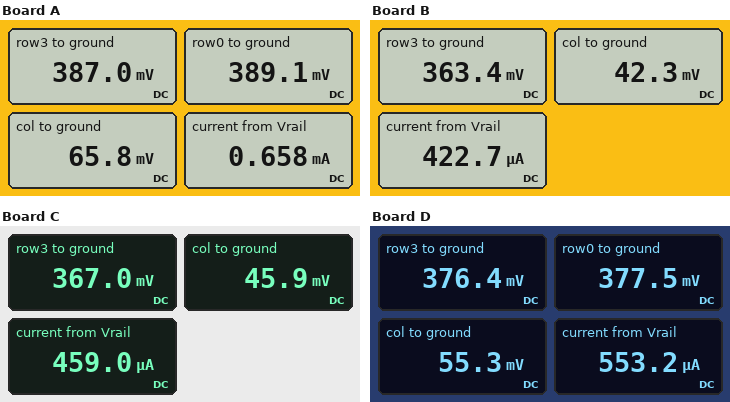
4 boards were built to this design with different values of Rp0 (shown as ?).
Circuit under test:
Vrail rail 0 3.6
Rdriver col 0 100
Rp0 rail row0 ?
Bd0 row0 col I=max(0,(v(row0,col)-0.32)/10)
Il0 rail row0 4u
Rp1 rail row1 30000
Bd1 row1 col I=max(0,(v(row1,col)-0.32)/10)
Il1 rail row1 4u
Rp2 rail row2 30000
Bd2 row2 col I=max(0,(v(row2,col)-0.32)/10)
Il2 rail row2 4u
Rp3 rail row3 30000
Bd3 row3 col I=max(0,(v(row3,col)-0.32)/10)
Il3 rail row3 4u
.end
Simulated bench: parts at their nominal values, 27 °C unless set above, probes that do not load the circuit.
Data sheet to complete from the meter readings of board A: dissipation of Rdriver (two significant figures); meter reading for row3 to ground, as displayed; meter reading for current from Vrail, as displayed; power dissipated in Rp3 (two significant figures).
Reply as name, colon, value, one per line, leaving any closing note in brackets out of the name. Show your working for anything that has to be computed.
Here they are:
dissipation of Rdriver: (65.8 mV)^2 / 100 Ω = 43 µW
meter reading for row3 to ground, as displayed: 387.0 mV
meter reading for current from Vrail, as displayed: 0.658 mA
power dissipated in Rp3: (3.6 V - 387 mV)^2 / 30 kΩ = 340 µW
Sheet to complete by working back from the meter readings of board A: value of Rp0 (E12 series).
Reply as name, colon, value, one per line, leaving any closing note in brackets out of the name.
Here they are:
value of Rp0: 10 kΩ
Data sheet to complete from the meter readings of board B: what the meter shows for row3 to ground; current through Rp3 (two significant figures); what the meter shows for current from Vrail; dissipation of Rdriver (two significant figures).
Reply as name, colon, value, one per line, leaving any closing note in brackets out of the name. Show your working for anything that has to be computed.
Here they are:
what the meter shows for row3 to ground: 363.4 mV
current through Rp3: (3.6 V - 363.4 mV) / 30 kΩ = 110 µA
what the meter shows for current from Vrail: 422.7 µA
dissipation of Rdriver: (42.3 mV)^2 / 100 Ω = 18 µW
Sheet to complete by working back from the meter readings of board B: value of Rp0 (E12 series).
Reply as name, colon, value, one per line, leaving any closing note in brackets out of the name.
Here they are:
value of Rp0: 39 kΩ
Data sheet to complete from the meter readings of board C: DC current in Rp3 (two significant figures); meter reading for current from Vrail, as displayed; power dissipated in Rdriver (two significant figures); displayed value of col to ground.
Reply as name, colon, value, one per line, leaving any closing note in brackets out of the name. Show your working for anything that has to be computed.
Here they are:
DC current in Rp3: (3.6 V - 367 mV) / 30 kΩ = 110 µA
meter reading for current from Vrail, as displayed: 459.0 µA
power dissipated in Rdriver: (45.9 mV)^2 / 100 Ω = 21 µW
displayed value of col to ground: 45.9 mV
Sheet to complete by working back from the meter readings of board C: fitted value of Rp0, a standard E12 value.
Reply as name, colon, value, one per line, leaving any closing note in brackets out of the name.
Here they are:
fitted value of Rp0, a standard E12 value: 27 kΩ
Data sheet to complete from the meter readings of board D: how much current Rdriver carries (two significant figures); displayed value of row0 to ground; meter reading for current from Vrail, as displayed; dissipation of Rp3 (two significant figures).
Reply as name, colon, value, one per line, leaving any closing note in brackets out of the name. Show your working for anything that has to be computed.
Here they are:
how much current Rdriver carries: (55.3 mV) / 100 Ω = 550 µA
displayed value of row0 to ground: 377.5 mV
meter reading for current from Vrail, as displayed: 553.2 µA
dissipation of Rp3: (3.6 V - 376.4 mV)^2 / 30 kΩ = 350 µW
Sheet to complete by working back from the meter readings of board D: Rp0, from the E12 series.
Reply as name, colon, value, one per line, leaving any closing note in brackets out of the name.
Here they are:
Rp0, from the E12 series: 15 kΩ
